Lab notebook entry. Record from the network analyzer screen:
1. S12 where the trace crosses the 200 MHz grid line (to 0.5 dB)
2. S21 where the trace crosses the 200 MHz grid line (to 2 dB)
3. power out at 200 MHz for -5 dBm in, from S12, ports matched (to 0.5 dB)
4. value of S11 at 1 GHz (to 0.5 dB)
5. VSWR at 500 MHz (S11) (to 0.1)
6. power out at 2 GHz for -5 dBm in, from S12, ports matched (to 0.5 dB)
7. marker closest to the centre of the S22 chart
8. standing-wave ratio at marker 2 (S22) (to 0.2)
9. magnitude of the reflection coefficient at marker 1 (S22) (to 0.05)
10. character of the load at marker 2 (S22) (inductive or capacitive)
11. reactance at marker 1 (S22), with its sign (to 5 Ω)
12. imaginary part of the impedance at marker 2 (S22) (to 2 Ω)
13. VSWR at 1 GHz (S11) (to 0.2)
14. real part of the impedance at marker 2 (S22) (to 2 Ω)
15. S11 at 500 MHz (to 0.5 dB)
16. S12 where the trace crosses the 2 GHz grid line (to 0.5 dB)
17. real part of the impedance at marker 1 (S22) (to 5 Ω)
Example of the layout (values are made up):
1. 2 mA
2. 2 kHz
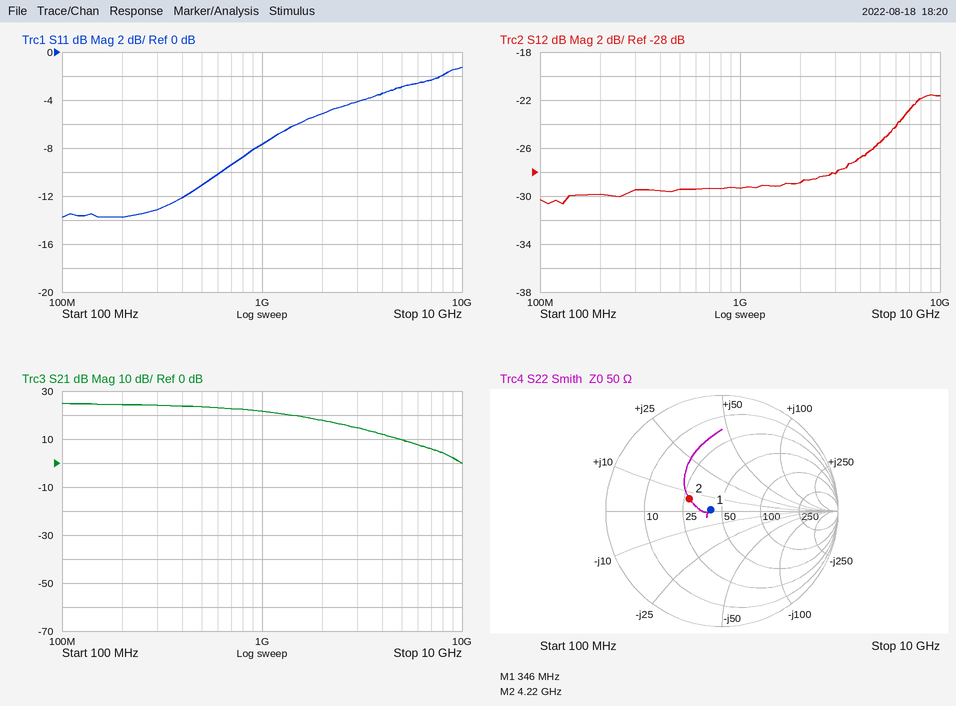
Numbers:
1. -30.0 dB
2. 24 dB
3. -35.0 dBm
4. -7.5 dB
5. 1.8
6. -34.0 dBm
7. marker 1
8. 1.8
9. 0.10
10. inductive
11. 0 Ω
12. +6 Ω
13. 2.4
14. 28 Ω
15. -11.0 dB
16. -29.0 dB
17. 40 Ω
